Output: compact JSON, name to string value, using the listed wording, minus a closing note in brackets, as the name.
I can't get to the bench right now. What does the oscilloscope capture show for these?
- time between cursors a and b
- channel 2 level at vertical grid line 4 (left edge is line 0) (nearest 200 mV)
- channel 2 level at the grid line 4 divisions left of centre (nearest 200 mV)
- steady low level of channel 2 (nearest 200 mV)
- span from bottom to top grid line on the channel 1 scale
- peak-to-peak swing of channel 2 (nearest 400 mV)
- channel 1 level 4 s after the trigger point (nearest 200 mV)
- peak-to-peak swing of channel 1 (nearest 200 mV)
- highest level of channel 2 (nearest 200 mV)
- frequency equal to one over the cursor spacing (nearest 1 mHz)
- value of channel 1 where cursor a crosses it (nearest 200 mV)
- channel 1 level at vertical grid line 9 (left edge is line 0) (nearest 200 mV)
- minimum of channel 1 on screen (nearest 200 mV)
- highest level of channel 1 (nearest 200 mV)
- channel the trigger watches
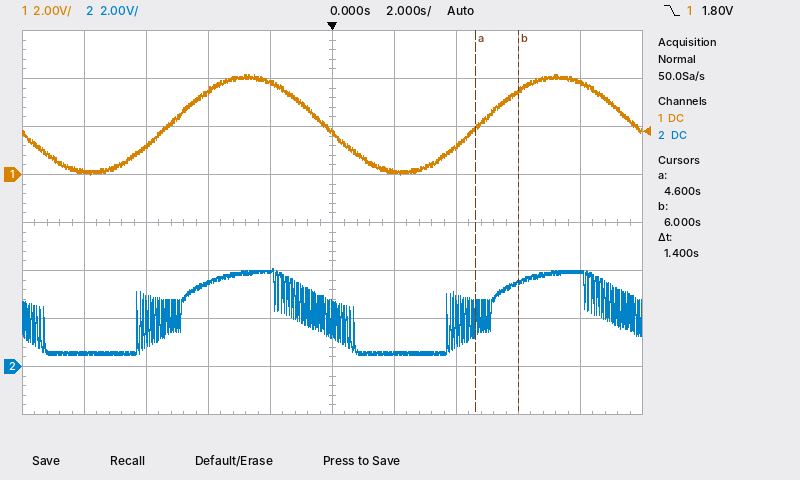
{"time between cursors a and b": "1.4 s", "channel 2 level at vertical grid line 4 (left edge is line 0)": "4.0 V", "channel 2 level at the grid line 4 divisions left of centre": "600 mV", "steady low level of channel 2": "600 mV", "span from bottom to top grid line on the channel 1 scale": "16 V", "peak-to-peak swing of channel 2": "3.6 V", "channel 1 level 4 s after the trigger point": "1.2 V", "peak-to-peak swing of channel 1": "4.2 V", "highest level of channel 2": "4.0 V", "frequency equal to one over the cursor spacing": "714 mHz", "value of channel 1 where cursor a crosses it": "2.0 V", "channel 1 level at vertical grid line 9 (left edge is line 0)": "3.8 V", "minimum of channel 1 on screen": "0.0 V", "highest level of channel 1": "4.2 V", "channel the trigger watches": "channel 1"}
